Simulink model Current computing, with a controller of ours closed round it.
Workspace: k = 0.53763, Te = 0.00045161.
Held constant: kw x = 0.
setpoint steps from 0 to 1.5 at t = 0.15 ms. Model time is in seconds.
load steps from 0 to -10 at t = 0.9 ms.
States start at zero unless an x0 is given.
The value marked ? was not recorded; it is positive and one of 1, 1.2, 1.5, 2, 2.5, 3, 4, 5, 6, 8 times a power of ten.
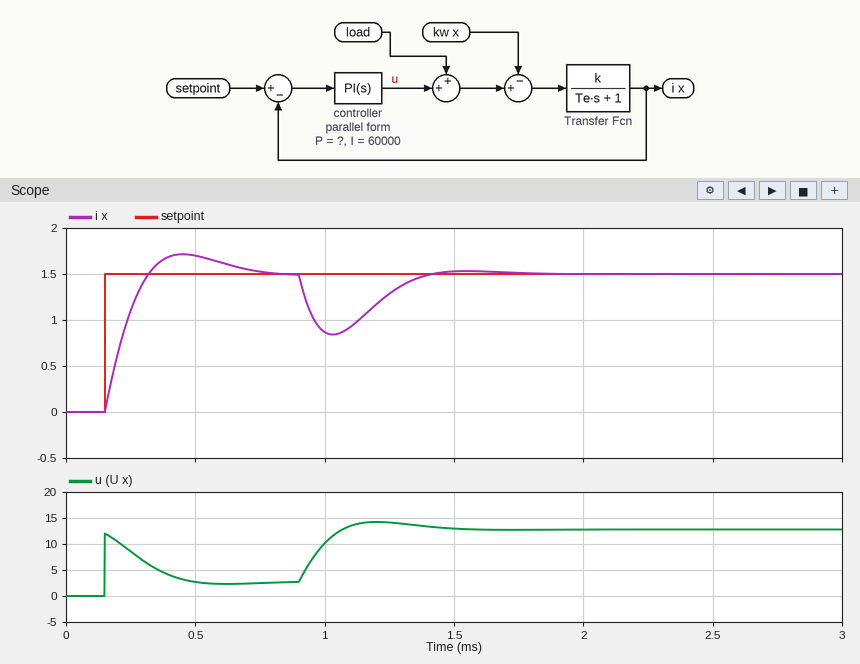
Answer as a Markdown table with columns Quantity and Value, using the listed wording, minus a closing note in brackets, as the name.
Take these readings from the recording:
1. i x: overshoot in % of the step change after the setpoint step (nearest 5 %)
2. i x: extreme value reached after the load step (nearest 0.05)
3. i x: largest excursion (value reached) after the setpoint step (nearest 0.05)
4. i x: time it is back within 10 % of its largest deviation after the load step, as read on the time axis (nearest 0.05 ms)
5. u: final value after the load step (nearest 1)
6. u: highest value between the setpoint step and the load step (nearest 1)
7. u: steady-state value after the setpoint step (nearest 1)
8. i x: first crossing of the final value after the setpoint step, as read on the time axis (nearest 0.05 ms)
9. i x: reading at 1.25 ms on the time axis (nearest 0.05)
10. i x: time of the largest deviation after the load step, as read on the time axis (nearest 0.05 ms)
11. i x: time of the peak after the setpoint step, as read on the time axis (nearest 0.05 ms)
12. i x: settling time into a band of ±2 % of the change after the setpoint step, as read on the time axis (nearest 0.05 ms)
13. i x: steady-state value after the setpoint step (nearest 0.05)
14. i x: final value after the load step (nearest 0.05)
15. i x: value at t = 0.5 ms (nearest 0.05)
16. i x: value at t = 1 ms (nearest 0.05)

| Quantity | Value |
|---|---|
| i x: overshoot in % of the step change after the setpoint step | 15 % |
| i x: extreme value reached after the load step | 0.85 |
| i x: largest excursion (value reached) after the setpoint step | 1.70 |
| i x: time it is back within 10 % of its largest deviation after the load step, as read on the time axis | 1.35 ms |
| u: final value after the load step | 13 |
| u: highest value between the setpoint step and the load step | 12 |
| u: steady-state value after the setpoint step | 3 |
| i x: first crossing of the final value after the setpoint step, as read on the time axis | 0.30 ms |
| i x: reading at 1.25 ms on the time axis | 1.30 |
| i x: time of the largest deviation after the load step, as read on the time axis | 1.05 ms |
| i x: time of the peak after the setpoint step, as read on the time axis | 0.45 ms |
| i x: settling time into a band of ±2 % of the change after the setpoint step, as read on the time axis | 0.75 ms |
| i x: steady-state value after the setpoint step | 1.50 |
| i x: final value after the load step | 1.50 |
| i x: value at t = 0.5 ms | 1.70 |
| i x: value at t = 1 ms | 0.85 |
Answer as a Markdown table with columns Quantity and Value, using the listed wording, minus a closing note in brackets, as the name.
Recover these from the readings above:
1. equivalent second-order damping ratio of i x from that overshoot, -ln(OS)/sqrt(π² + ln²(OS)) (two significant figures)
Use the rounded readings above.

| Quantity | Value |
|---|---|
| equivalent second-order damping ratio of i x from that overshoot, -ln(OS)/sqrt(π² + ln²(OS)) | 0.52 |
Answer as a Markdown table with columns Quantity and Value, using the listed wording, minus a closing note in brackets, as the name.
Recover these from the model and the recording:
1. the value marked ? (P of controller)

| Quantity | Value |
|---|---|
| the value marked ? | 8 |
